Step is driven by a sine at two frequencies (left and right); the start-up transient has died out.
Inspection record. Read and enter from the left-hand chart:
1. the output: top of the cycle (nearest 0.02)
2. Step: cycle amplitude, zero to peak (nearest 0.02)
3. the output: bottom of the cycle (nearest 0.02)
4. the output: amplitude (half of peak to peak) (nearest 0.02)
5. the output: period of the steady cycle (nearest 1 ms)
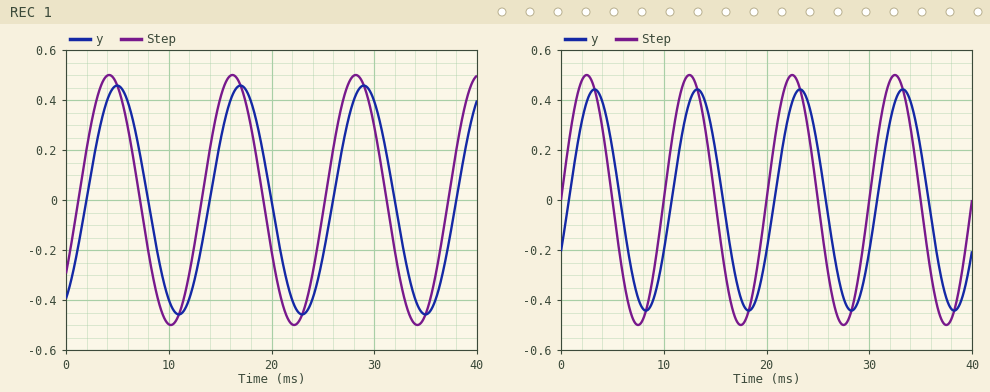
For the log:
0.46
0.50
-0.46
0.46
12 ms
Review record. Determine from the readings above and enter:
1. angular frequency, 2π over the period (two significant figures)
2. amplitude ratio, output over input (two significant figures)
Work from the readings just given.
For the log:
0.52 rad/ms
0.92
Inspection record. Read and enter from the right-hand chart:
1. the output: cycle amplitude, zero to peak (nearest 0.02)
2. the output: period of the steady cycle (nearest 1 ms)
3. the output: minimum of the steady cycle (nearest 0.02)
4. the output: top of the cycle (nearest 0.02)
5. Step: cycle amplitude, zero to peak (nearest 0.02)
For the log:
0.44
10 ms
-0.44
0.44
0.50
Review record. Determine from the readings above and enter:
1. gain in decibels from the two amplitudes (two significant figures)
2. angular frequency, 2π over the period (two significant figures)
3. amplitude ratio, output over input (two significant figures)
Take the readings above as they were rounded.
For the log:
-1.1 dB
0.63 rad/ms
0.88
